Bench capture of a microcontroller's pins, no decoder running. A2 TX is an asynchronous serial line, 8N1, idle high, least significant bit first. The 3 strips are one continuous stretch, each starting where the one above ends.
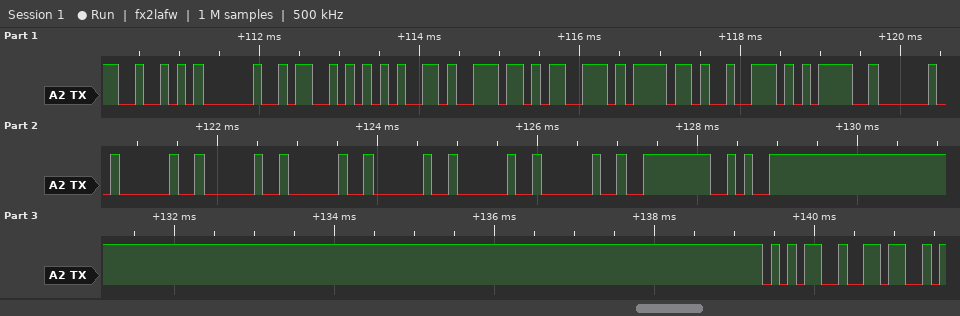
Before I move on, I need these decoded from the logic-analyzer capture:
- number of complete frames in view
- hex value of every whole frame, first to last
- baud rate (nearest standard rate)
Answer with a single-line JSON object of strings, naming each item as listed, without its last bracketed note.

{"number of complete frames in view": "20", "hex value of every whole frame, first to last": "0x52 0x20 0x53 0x65 0x6E 0x73 0x6F 0x72 0x3D 0x20 0x20 0x20 0x20 0x20 0x20 0x20 0xFE 0xCA 0x35 0x36", "baud rate": "9600 baud"}
